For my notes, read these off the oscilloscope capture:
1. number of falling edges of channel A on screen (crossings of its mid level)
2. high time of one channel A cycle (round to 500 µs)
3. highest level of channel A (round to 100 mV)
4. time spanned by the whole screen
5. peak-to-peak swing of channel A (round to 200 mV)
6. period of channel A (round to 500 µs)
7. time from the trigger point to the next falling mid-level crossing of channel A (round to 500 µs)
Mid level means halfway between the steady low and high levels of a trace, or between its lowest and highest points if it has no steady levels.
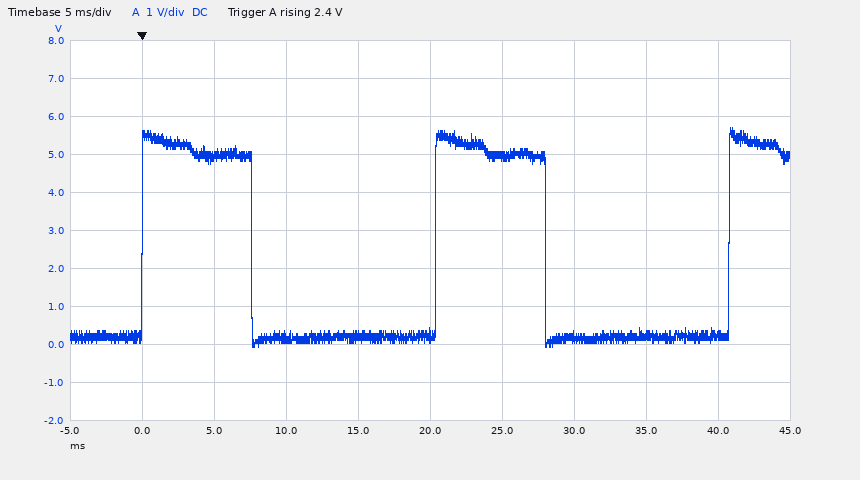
2
7.5 ms
5.7 V
50 ms
5.8 V
20.5 ms
7.5 ms
